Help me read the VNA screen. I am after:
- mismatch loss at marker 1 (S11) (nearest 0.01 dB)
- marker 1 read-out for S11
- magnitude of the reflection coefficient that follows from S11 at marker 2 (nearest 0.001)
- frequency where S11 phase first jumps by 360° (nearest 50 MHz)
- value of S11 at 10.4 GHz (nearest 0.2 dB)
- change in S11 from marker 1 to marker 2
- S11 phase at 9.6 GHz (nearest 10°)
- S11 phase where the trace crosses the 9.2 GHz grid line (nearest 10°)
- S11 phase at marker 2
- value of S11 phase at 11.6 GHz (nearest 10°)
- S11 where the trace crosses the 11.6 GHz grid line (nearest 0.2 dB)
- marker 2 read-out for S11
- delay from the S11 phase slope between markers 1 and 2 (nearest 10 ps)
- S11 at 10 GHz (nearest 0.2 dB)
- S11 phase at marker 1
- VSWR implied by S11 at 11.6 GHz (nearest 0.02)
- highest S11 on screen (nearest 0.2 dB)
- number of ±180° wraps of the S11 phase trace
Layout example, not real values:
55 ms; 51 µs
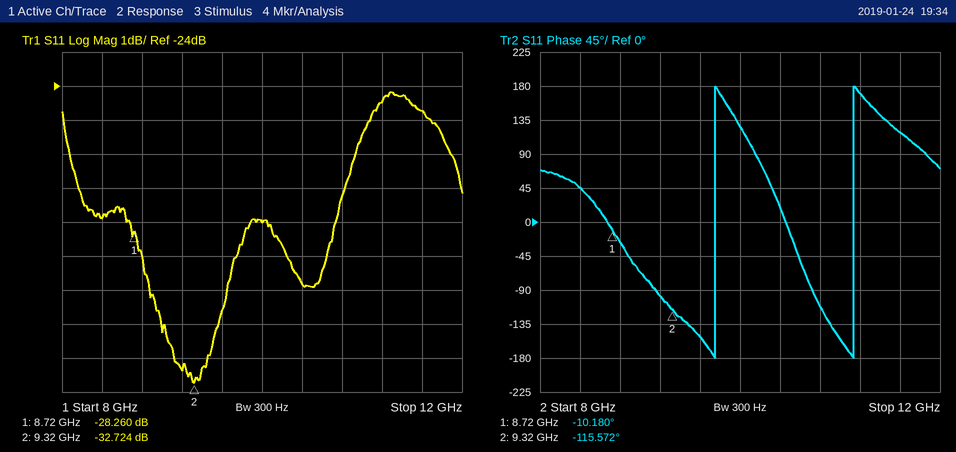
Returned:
0.01 dB; -28.260 dB; 0.023; 9.75 GHz; -29.8 dB; -4.464 dB; -150°; -100°; -115.572°; 120°; -24.8 dB; -32.724 dB; 490 ps; -28.0 dB; -10.180°; 1.12; -24.2 dB; 2
